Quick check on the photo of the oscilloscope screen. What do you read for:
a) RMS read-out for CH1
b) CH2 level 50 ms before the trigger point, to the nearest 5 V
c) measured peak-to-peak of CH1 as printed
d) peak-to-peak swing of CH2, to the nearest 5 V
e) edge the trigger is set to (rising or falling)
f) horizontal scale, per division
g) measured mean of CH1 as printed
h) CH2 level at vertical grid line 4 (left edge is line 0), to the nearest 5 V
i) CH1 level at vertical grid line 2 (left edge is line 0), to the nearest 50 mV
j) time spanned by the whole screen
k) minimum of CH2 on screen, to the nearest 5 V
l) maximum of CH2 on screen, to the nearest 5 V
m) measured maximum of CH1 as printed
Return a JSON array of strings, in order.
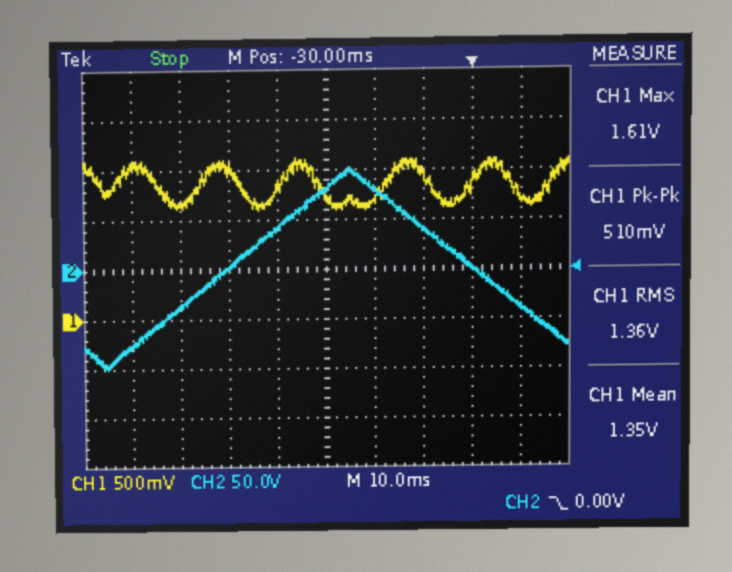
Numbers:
["1.36 V", "0 V", "510 mV", "200 V", "falling", "10 ms", "1.35 V", "40 V", "1.15 V", "100 ms", "-100 V", "100 V", "1.61 V"]
